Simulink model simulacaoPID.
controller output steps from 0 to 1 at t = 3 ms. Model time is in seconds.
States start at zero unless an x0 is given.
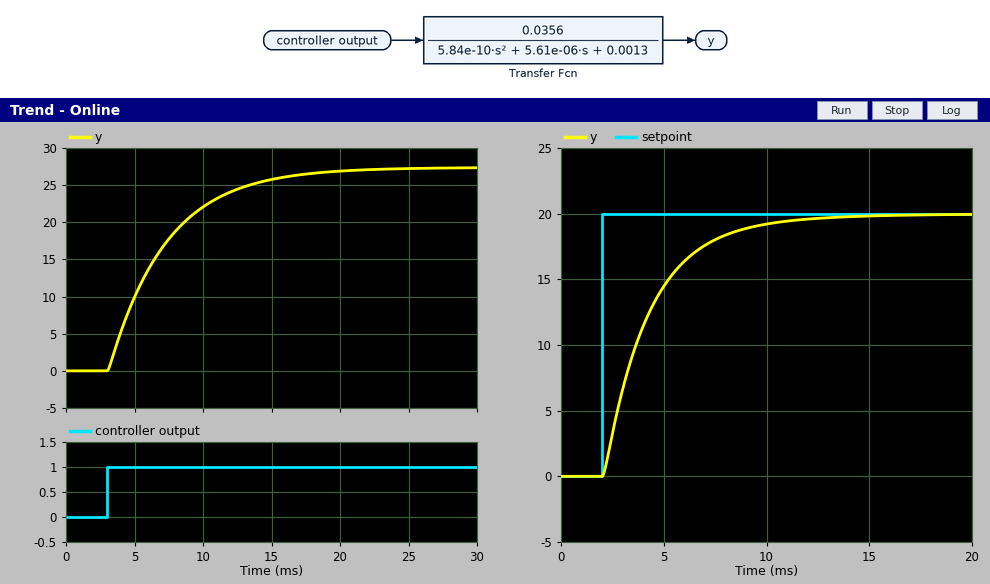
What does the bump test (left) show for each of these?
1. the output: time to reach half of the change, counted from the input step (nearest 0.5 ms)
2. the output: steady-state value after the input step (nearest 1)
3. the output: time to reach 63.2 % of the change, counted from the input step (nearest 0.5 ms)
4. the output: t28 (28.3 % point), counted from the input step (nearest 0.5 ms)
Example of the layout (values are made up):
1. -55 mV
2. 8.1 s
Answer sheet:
1. 3.0 ms
2. 27
3. 4.5 ms
4. 1.5 ms
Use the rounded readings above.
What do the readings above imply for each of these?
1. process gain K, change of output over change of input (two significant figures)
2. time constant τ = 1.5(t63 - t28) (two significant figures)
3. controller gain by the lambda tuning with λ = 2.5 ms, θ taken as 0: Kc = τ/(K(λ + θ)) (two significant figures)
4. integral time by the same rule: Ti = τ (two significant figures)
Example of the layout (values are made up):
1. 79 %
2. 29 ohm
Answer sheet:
1. 27
2. 4.5 ms
3. 0.067
4. 4.5 ms
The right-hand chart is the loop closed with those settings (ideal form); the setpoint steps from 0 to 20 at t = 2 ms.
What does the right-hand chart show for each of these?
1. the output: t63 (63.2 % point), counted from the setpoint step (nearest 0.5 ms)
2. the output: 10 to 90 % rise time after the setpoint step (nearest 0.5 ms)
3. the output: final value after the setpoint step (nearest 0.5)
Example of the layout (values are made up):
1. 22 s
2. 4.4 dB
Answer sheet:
1. 2.5 ms
2. 5.0 ms
3. 20.0
